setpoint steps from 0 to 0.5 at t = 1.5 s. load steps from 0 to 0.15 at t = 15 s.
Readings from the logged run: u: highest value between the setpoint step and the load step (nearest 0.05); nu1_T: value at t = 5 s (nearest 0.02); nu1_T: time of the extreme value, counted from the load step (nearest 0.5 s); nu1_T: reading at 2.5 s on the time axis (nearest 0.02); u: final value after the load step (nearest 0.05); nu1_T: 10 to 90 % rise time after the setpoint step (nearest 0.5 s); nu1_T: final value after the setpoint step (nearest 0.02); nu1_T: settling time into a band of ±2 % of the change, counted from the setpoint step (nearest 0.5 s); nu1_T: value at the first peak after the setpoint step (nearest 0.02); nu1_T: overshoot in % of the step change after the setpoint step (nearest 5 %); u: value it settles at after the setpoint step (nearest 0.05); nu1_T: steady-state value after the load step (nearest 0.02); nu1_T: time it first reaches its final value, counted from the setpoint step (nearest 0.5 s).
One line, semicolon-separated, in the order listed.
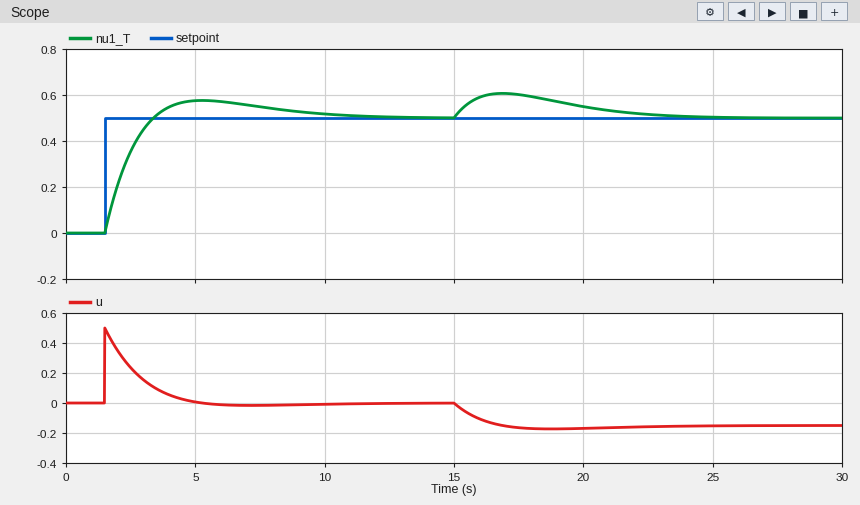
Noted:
0.50; 0.58; 2.0 s; 0.36; -0.15; 1.5 s; 0.50; 9.5 s; 0.58; 15 %; 0.00; 0.50; 2.0 s
